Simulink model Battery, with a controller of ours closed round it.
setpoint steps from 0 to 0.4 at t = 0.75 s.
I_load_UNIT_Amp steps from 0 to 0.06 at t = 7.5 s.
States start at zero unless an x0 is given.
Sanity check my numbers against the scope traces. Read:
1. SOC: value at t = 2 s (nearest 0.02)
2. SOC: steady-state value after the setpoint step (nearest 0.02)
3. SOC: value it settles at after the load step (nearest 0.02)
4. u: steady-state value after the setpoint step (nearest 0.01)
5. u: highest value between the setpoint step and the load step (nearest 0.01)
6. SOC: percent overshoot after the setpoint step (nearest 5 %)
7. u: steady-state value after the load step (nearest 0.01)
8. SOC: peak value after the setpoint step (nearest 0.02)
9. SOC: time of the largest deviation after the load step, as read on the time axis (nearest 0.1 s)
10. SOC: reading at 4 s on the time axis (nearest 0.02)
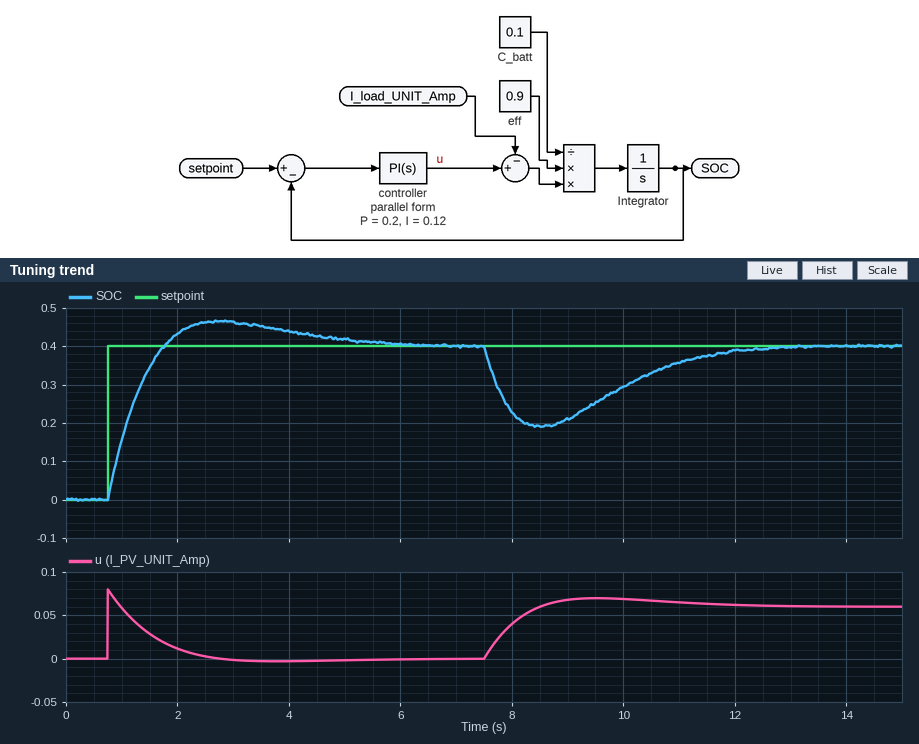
0.44
0.40
0.40
0.00
0.08
15 %
0.06
0.46
8.5 s
0.44
